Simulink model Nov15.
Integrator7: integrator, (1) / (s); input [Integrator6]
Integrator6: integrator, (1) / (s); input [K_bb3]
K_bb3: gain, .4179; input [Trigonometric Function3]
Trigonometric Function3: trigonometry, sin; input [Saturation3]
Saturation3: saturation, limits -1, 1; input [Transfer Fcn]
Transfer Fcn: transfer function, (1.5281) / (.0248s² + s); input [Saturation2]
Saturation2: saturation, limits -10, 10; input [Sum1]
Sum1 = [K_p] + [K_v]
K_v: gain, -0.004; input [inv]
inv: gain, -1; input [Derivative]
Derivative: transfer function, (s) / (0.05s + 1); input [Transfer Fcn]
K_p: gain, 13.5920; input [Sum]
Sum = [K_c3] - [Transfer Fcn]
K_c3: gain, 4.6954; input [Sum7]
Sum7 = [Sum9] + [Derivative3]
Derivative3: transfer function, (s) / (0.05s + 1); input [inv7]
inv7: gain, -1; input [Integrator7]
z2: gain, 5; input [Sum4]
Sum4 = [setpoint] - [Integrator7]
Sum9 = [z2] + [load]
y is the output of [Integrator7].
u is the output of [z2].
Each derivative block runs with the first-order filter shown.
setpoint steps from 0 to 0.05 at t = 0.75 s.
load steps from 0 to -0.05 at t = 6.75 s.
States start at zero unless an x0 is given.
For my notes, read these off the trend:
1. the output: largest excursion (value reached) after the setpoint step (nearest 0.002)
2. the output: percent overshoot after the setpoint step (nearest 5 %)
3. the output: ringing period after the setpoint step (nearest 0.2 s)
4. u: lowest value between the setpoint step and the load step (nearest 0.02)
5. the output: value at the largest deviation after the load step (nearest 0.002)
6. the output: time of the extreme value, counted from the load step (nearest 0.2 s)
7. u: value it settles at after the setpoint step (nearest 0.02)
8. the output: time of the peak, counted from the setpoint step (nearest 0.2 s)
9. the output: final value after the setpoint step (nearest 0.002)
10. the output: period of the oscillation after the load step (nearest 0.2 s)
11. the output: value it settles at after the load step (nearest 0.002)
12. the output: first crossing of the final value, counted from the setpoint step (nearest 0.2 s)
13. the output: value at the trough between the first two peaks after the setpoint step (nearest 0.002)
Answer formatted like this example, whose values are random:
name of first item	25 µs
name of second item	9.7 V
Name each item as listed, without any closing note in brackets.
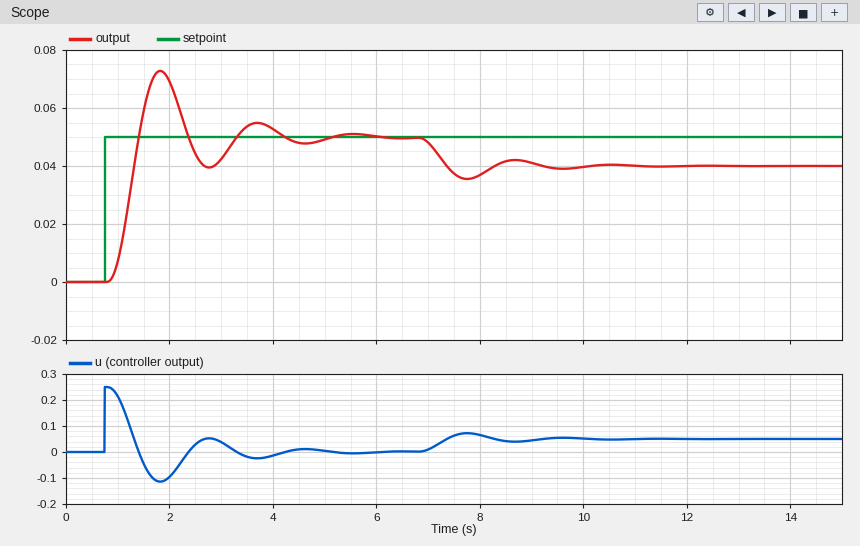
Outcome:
the output: largest excursion (value reached) after the setpoint step	0.072
the output: percent overshoot after the setpoint step	45 %
the output: ringing period after the setpoint step	1.8 s
u: lowest value between the setpoint step and the load step	-0.12
the output: value at the largest deviation after the load step	0.036
the output: time of the extreme value, counted from the load step	1.0 s
u: value it settles at after the setpoint step	0.00
the output: time of the peak, counted from the setpoint step	1.0 s
the output: final value after the setpoint step	0.050
the output: period of the oscillation after the load step	1.8 s
the output: value it settles at after the load step	0.040
the output: first crossing of the final value, counted from the setpoint step	0.6 s
the output: value at the trough between the first two peaks after the setpoint step	0.040
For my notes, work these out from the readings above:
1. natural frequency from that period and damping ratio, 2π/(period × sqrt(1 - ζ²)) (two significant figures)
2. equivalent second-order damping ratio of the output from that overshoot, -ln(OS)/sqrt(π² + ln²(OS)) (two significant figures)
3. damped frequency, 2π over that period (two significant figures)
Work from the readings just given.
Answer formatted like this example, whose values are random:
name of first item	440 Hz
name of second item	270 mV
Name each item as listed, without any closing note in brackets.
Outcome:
natural frequency from that period and damping ratio, 2π/(period × sqrt(1 - ζ²))	3.6 rad/s
equivalent second-order damping ratio of the output from that overshoot, -ln(OS)/sqrt(π² + ln²(OS))	0.25
damped frequency, 2π over that period	3.5 rad/s
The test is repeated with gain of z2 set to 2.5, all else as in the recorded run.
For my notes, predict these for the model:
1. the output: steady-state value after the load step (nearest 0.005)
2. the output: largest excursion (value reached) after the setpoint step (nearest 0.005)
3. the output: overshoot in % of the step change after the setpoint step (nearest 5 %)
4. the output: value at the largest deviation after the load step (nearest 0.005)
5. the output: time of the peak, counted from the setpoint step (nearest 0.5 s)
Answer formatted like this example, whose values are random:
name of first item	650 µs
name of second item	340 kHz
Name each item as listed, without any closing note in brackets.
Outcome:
the output: steady-state value after the load step	0.030
the output: largest excursion (value reached) after the setpoint step	0.060
the output: overshoot in % of the step change after the setpoint step	25 %
the output: value at the largest deviation after the load step	0.025
the output: time of the peak, counted from the setpoint step	1.5 s
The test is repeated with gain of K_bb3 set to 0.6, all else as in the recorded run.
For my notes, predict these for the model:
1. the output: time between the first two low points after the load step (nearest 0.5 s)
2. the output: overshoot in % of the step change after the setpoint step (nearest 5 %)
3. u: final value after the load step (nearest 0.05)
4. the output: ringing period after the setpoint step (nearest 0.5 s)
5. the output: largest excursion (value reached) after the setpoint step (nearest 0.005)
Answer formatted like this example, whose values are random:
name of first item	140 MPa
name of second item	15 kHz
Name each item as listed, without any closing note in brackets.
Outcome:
the output: time between the first two low points after the load step	1.5 s
the output: overshoot in % of the step change after the setpoint step	40 %
u: final value after the load step	0.05
the output: ringing period after the setpoint step	1.5 s
the output: largest excursion (value reached) after the setpoint step	0.070
